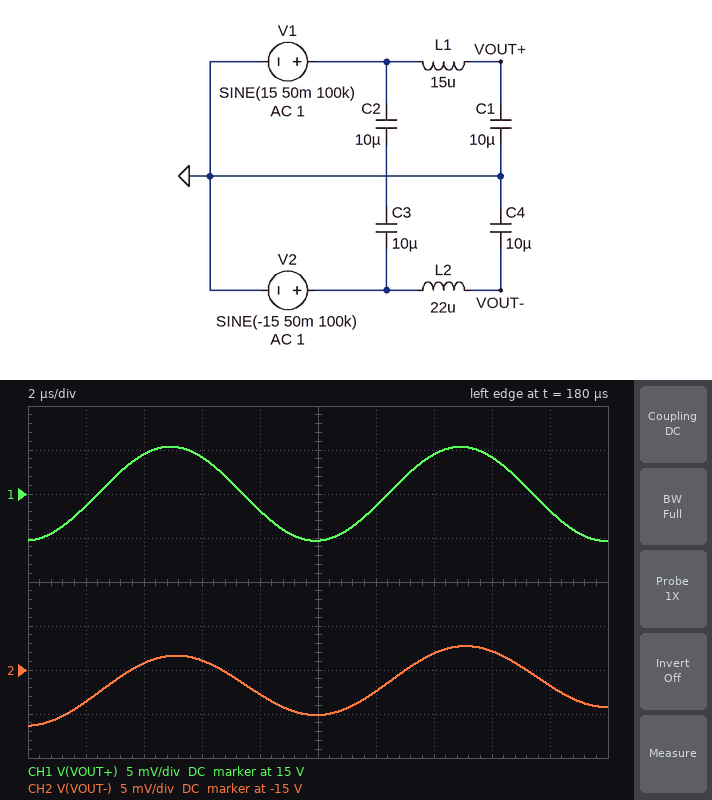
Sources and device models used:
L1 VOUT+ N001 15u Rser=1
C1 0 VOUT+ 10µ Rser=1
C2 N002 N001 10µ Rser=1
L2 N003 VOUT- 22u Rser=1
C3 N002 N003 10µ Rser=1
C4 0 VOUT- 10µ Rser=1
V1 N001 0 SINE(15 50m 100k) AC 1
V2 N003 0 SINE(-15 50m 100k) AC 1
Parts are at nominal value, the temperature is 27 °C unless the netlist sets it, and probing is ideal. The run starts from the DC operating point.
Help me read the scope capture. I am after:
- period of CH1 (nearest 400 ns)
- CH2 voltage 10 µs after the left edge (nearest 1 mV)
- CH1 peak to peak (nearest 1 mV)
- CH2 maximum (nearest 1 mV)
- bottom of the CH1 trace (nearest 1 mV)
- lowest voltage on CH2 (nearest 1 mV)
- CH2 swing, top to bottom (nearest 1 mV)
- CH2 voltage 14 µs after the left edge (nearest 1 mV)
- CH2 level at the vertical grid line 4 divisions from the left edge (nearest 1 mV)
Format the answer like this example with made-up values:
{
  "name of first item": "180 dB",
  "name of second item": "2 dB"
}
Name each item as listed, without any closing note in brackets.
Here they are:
{
  "period of CH1": "10.0 µs",
  "CH2 voltage 10 µs after the left edge": "-15.005 V",
  "CH1 peak to peak": "11 mV",
  "CH2 maximum": "-14.997 V",
  "bottom of the CH1 trace": "14.995 V",
  "lowest voltage on CH2": "-15.006 V",
  "CH2 swing, top to bottom": "9 mV",
  "CH2 voltage 14 µs after the left edge": "-14.998 V",
  "CH2 level at the vertical grid line 4 divisions from the left edge": "-15.003 V"
}
